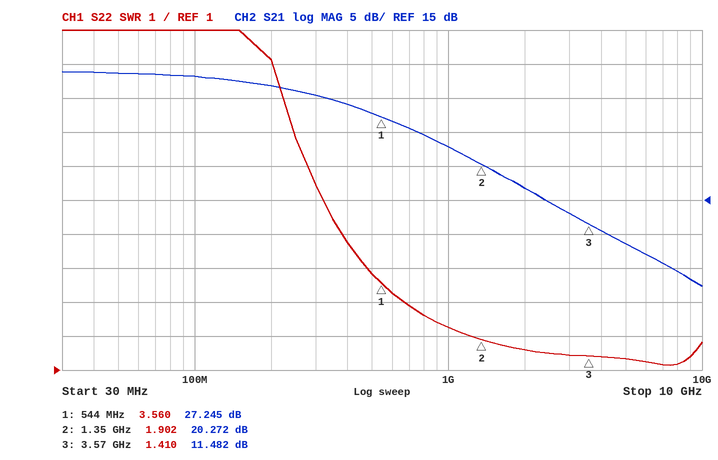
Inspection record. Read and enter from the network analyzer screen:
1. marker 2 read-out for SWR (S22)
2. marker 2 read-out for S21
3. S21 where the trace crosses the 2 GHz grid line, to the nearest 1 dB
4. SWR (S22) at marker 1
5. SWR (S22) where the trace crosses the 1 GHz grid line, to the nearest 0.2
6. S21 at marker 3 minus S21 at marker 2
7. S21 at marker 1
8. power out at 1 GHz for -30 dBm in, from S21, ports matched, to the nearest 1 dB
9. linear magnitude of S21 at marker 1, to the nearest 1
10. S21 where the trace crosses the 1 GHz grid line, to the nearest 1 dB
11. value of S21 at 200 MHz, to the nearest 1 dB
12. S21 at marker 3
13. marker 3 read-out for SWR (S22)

1.902
20.272 dB
17 dB
3.560
2.2
-8.790 dB
27.245 dB
-7 dBm
23
23 dB
32 dB
11.482 dB
1.410
